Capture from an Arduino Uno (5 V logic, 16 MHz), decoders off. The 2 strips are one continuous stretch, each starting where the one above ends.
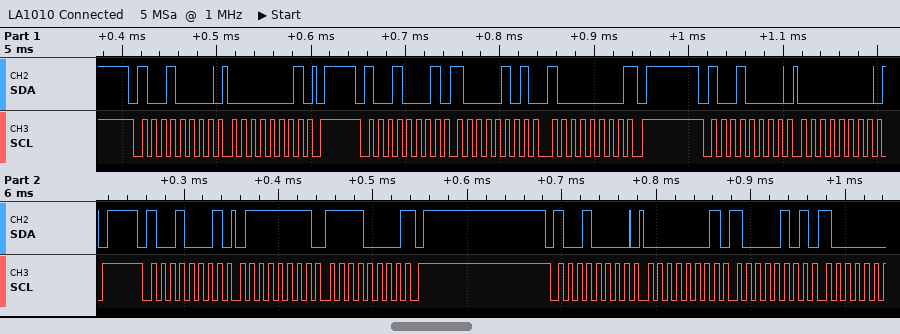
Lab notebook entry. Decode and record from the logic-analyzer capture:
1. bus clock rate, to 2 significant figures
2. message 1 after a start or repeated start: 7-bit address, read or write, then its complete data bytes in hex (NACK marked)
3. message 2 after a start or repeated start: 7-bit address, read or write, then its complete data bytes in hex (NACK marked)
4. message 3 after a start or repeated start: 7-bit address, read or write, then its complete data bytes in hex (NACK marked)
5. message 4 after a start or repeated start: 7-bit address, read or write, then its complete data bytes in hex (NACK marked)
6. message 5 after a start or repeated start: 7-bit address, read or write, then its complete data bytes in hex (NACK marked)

100 kHz
0x48 write: 01
0x48 read: 85 80 NACK
0x48 write: 00
0x48 read: 7F F0 NACK
0x48 write: 01 85
